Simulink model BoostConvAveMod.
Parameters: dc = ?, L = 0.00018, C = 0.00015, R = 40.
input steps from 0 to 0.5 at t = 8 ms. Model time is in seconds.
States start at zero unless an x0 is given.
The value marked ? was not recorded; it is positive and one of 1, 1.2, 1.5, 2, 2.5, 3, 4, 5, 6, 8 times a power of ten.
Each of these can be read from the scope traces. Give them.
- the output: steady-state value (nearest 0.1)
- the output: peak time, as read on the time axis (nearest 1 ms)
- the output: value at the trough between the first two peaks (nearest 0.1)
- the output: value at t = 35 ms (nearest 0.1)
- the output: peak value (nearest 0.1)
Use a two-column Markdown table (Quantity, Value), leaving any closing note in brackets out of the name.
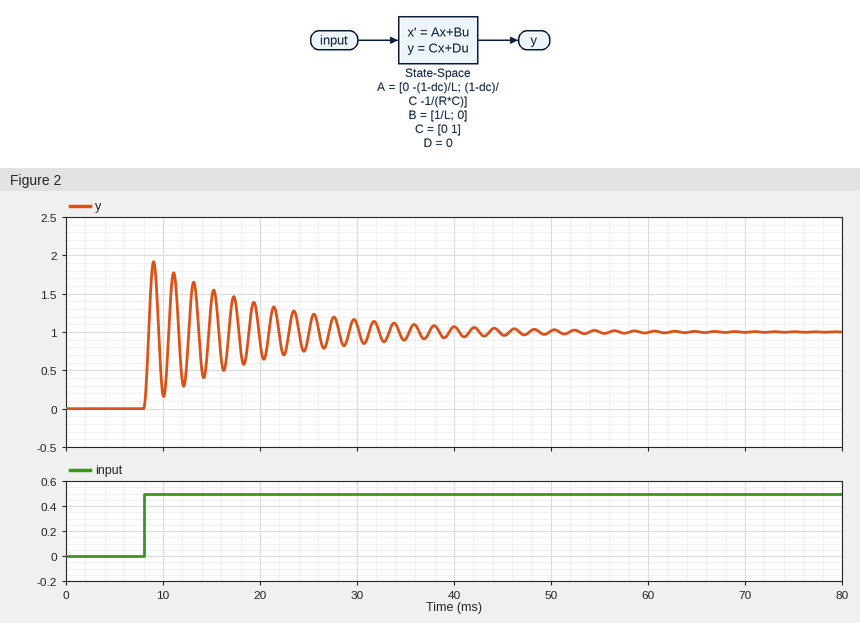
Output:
| Quantity | Value |
|---|---|
| the output: steady-state value | 1.0 |
| the output: peak time, as read on the time axis | 9 ms |
| the output: value at the trough between the first two peaks | 0.2 |
| the output: value at t = 35 ms | 0.9 |
| the output: peak value | 1.9 |
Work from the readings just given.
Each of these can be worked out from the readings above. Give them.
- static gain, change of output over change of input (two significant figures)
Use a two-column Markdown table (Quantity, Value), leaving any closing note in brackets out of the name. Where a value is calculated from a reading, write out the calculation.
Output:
| Quantity | Value |
|---|---|
| static gain, change of output over change of input | (1 - 0) / (0.5 - 0) = 2.0 |
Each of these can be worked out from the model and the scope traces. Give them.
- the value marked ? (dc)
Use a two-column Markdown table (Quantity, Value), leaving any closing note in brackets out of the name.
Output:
| Quantity | Value |
|---|---|
| the value marked ? | 0.5 |
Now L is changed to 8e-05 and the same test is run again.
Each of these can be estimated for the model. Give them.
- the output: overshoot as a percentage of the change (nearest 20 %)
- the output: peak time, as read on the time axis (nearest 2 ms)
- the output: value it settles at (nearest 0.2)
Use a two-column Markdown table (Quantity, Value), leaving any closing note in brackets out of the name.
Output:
| Quantity | Value |
|---|---|
| the output: overshoot as a percentage of the change | 100 % |
| the output: peak time, as read on the time axis | 8 ms |
| the output: value it settles at | 1.0 |
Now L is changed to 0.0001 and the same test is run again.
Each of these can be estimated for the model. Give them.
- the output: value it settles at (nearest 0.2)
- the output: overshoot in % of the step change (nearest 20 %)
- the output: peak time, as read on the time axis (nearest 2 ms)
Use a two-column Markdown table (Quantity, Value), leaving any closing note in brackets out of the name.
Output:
| Quantity | Value |
|---|---|
| the output: value it settles at | 1.0 |
| the output: overshoot in % of the step change | 100 % |
| the output: peak time, as read on the time axis | 8 ms |
